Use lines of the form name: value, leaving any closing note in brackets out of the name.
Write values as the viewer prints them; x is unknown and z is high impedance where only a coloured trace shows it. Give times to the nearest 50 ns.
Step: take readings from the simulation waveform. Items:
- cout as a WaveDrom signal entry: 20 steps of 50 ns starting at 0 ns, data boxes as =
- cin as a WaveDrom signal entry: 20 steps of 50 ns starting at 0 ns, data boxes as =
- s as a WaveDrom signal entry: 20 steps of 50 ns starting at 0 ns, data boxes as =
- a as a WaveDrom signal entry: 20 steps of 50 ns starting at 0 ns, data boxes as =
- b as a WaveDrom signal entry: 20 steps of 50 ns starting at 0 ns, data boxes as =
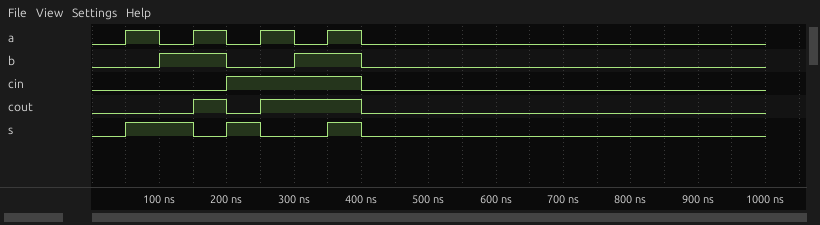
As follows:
cout as a WaveDrom signal entry: 20 steps of 50 ns starting at 0 ns, data boxes as =: {name: 'cout', wave: '0..101..0...........'}
cin as a WaveDrom signal entry: 20 steps of 50 ns starting at 0 ns, data boxes as =: {name: 'cin', wave: '0...1...0...........'}
s as a WaveDrom signal entry: 20 steps of 50 ns starting at 0 ns, data boxes as =: {name: 's', wave: '01.010.10...........'}
a as a WaveDrom signal entry: 20 steps of 50 ns starting at 0 ns, data boxes as =: {name: 'a', wave: '010101010...........'}
b as a WaveDrom signal entry: 20 steps of 50 ns starting at 0 ns, data boxes as =: {name: 'b', wave: '0.1.0.1.0...........'}
